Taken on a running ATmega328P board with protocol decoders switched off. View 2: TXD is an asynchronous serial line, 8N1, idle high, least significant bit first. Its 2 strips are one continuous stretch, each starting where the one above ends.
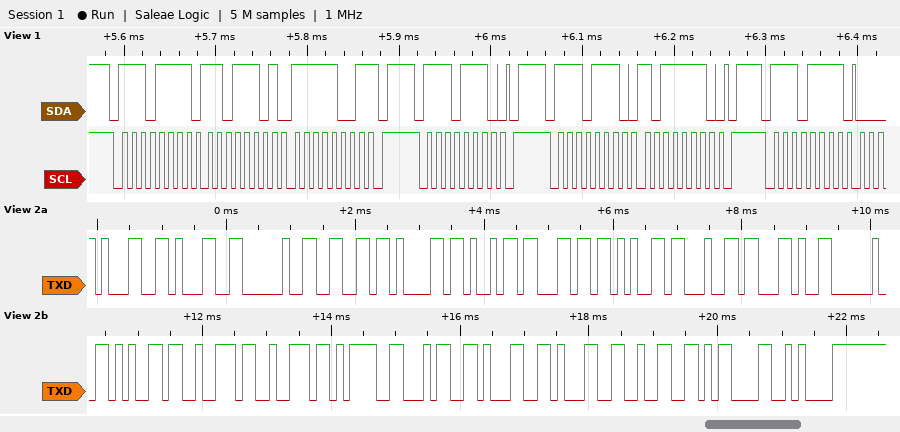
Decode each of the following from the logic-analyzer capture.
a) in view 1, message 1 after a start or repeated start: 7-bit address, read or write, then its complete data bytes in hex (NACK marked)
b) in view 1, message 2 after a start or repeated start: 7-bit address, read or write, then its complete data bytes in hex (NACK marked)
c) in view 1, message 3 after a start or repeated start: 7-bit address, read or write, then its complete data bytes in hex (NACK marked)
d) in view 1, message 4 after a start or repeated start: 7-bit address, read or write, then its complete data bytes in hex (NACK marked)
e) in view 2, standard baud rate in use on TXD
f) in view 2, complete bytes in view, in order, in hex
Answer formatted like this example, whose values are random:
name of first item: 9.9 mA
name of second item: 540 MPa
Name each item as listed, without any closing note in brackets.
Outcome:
in view 1, message 1 after a start or repeated start: 7-bit address, read or write, then its complete data bytes in hex: 0x77 read: DD F9 NACK
in view 1, message 2 after a start or repeated start: 7-bit address, read or write, then its complete data bytes in hex: 0x77 write
in view 1, message 3 after a start or repeated start: 7-bit address, read or write, then its complete data bytes in hex: 0x77 write: BE
in view 1, message 4 after a start or repeated start: 7-bit address, read or write, then its complete data bytes in hex: 0x77 read
in view 2, standard baud rate in use on TXD: 9600 baud
in view 2, complete bytes in view, in order, in hex: 31 31 20 66 61 69 6C 65 64 2C 20 65 72 72 3D 34 31 31 32 0D 0A
